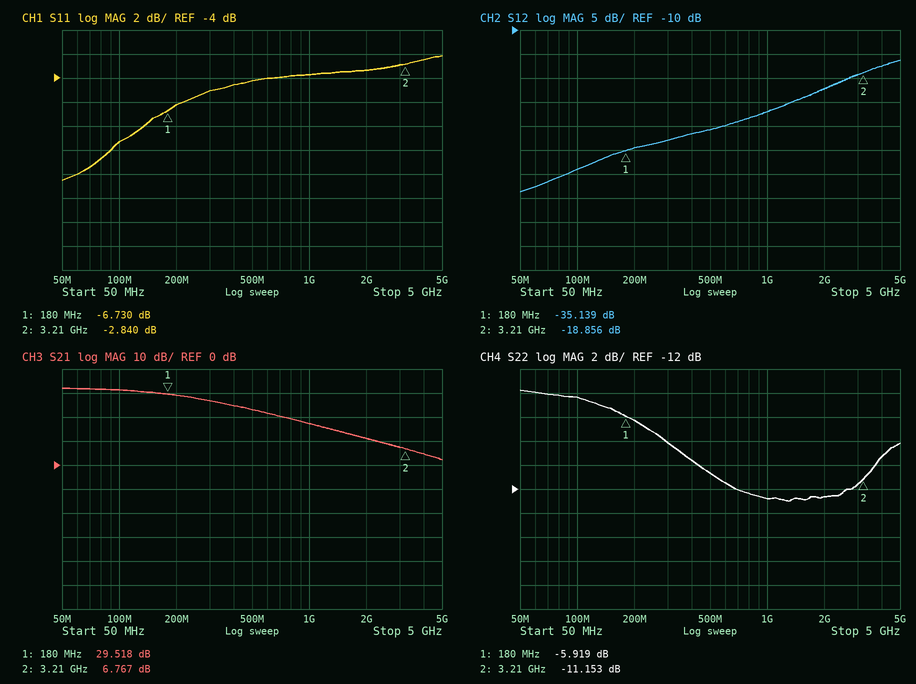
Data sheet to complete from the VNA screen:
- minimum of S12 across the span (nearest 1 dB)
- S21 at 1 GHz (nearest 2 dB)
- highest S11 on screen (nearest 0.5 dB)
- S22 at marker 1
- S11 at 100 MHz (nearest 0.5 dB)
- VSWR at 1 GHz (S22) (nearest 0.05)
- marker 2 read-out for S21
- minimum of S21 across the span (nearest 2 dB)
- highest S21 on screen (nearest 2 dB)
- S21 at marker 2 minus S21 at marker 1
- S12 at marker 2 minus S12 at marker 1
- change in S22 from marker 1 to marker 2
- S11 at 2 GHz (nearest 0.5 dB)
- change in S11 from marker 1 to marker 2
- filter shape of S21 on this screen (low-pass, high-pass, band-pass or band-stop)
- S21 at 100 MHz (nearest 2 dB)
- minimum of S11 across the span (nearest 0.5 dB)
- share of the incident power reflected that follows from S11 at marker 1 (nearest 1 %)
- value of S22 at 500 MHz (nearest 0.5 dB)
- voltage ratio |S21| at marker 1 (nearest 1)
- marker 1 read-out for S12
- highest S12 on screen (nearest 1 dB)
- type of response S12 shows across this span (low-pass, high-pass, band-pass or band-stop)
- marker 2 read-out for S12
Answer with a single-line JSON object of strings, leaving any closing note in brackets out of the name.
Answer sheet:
{"minimum of S12 across the span": "-44 dB", "S21 at 1 GHz": "18 dB", "highest S11 on screen": "-2.0 dB", "S22 at marker 1": "-5.919 dB", "S11 at 100 MHz": "-9.5 dB", "VSWR at 1 GHz (S22)": "1.60", "marker 2 read-out for S21": "6.767 dB", "minimum of S21 across the span": "2 dB", "highest S21 on screen": "32 dB", "S21 at marker 2 minus S21 at marker 1": "-22.751 dB", "S12 at marker 2 minus S12 at marker 1": "16.283 dB", "change in S22 from marker 1 to marker 2": "-5.234 dB", "S11 at 2 GHz": "-3.5 dB", "change in S11 from marker 1 to marker 2": "3.890 dB", "filter shape of S21 on this screen": "low-pass", "S21 at 100 MHz": "32 dB", "minimum of S11 across the span": "-12.5 dB", "share of the incident power reflected that follows from S11 at marker 1": "21 %", "value of S22 at 500 MHz": "-10.5 dB", "voltage ratio |S21| at marker 1": "30", "marker 1 read-out for S12": "-35.139 dB", "highest S12 on screen": "-16 dB", "type of response S12 shows across this span": "high-pass", "marker 2 read-out for S12": "-18.856 dB"}
